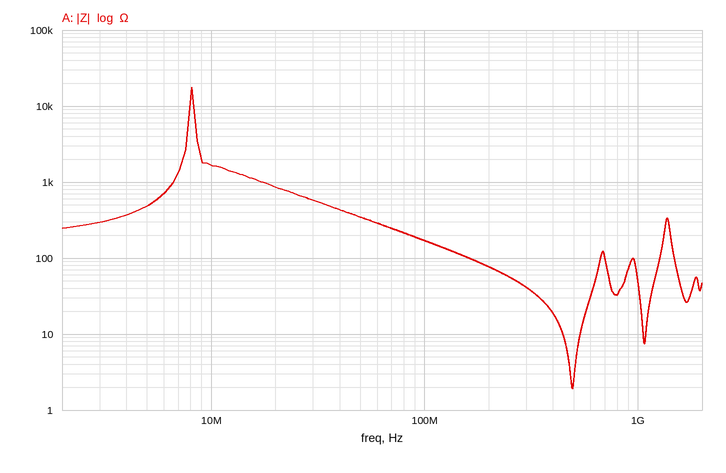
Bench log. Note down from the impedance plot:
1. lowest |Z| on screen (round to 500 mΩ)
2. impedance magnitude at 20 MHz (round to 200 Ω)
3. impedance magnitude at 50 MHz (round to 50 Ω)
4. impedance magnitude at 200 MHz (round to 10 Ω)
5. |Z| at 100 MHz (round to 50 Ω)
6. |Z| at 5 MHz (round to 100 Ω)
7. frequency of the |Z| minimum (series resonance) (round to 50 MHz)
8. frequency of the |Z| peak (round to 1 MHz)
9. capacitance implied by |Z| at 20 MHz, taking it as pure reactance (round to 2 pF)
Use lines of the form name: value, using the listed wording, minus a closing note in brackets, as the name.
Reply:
lowest |Z| on screen: 2.0 Ω
impedance magnitude at 20 MHz: 800 Ω
impedance magnitude at 50 MHz: 350 Ω
impedance magnitude at 200 MHz: 80 Ω
|Z| at 100 MHz: 150 Ω
|Z| at 5 MHz: 500 Ω
frequency of the |Z| minimum (series resonance): 500 MHz
frequency of the |Z| peak: 8 MHz
capacitance implied by |Z| at 20 MHz, taking it as pure reactance: 10 pF
